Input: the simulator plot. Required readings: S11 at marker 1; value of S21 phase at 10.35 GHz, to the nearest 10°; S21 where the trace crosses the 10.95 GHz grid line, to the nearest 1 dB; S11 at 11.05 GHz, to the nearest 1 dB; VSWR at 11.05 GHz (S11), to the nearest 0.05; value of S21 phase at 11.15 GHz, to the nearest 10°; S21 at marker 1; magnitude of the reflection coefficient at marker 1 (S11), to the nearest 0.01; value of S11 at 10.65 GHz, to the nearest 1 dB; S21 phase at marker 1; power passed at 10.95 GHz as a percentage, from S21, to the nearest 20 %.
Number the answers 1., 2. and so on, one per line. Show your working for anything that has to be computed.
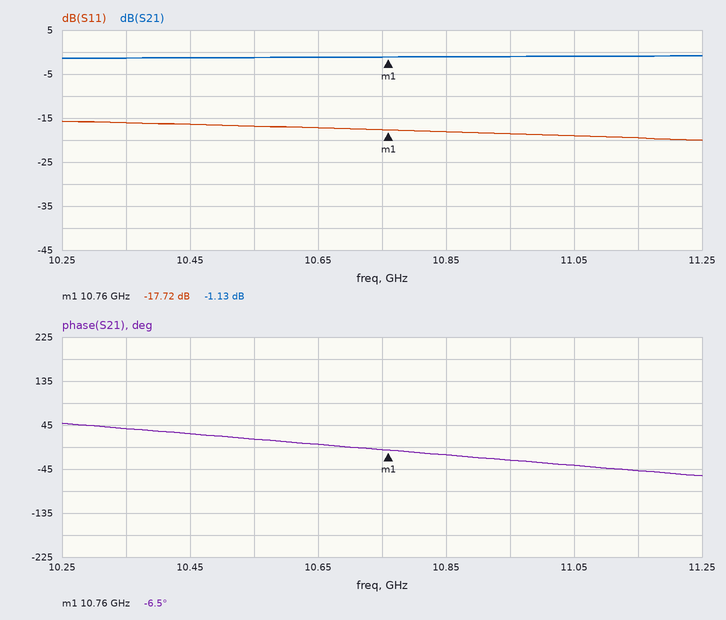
1. -17.72 dB
2. 40°
3. -1 dB
4. -19 dB
5. |Γ| = 10^(-19/20) = 0.1122; VSWR = (1 + 0.1122)/(1 − 0.1122) ≈ 1.25
6. -50°
7. -1.13 dB
8. 10^(-17.72/20) ≈ 0.13
9. -17 dB
10. -6.5°
11. 10^(-1/10) ≈ 79.4 %, so 80 % to the nearest 20 %
